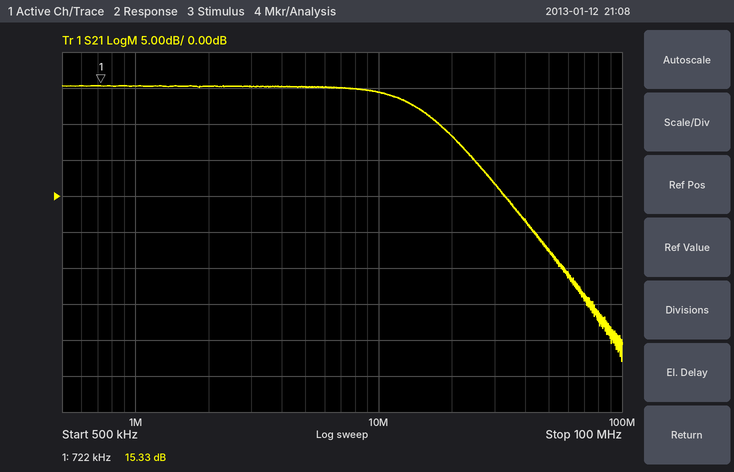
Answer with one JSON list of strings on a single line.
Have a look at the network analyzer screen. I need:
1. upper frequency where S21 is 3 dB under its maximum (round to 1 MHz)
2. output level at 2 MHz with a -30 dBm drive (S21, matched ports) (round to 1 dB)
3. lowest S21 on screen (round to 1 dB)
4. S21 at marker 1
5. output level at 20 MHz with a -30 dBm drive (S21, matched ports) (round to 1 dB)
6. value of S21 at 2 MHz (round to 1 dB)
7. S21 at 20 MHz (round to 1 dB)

["14 MHz", "-15 dBm", "-23 dB", "15.33 dB", "-22 dBm", "15 dB", "8 dB"]
